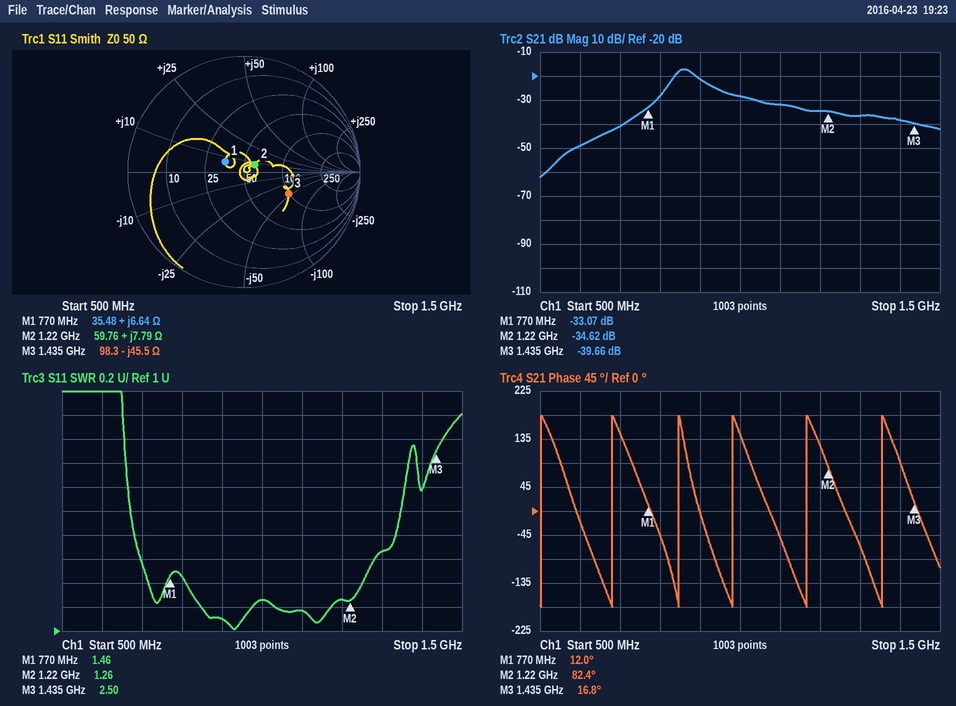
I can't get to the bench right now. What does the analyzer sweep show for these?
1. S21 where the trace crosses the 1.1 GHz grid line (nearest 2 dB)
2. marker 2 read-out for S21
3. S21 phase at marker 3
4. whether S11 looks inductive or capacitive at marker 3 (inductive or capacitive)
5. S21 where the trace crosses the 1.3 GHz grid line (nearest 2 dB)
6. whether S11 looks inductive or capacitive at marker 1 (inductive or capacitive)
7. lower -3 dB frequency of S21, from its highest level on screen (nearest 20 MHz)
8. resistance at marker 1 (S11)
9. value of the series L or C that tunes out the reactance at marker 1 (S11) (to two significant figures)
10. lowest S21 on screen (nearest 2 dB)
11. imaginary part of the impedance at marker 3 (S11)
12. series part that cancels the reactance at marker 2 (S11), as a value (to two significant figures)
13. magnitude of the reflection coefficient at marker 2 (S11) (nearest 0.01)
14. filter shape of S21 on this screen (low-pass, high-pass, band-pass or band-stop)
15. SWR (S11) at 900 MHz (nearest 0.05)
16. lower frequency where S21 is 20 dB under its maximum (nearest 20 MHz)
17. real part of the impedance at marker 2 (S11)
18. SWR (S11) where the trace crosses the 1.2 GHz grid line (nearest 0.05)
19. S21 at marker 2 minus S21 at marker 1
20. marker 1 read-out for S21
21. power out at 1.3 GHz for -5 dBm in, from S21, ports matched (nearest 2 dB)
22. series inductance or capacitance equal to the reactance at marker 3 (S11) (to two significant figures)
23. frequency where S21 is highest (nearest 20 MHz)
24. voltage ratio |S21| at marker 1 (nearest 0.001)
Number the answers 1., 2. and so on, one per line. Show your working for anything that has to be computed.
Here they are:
1. -32 dB
2. -34.62 dB
3. 16.8°
4. capacitive
5. -36 dB
6. inductive
7. 840 MHz
8. 35.48 Ω
9. C = 1/(2π × 770 MHz × 6.64 Ω) ≈ 31 pF
10. -62 dB
11. -45.5 Ω
12. C = 1/(2π × 1.22 GHz × 7.79 Ω) ≈ 17 pF
13. 0.11
14. band-pass
15. 1.10
16. 740 MHz
17. 59.76 Ω
18. 1.25
19. -34.62 − (-33.07) = -1.55 dB
20. -33.07 dB
21. -5 dBm + (-36 dB) = -42 dBm
22. C = 1/(2π × 1.435 GHz × 45.5 Ω) ≈ 2.4 pF
23. 860 MHz
24. 10^(-33.07/20) ≈ 0.022
